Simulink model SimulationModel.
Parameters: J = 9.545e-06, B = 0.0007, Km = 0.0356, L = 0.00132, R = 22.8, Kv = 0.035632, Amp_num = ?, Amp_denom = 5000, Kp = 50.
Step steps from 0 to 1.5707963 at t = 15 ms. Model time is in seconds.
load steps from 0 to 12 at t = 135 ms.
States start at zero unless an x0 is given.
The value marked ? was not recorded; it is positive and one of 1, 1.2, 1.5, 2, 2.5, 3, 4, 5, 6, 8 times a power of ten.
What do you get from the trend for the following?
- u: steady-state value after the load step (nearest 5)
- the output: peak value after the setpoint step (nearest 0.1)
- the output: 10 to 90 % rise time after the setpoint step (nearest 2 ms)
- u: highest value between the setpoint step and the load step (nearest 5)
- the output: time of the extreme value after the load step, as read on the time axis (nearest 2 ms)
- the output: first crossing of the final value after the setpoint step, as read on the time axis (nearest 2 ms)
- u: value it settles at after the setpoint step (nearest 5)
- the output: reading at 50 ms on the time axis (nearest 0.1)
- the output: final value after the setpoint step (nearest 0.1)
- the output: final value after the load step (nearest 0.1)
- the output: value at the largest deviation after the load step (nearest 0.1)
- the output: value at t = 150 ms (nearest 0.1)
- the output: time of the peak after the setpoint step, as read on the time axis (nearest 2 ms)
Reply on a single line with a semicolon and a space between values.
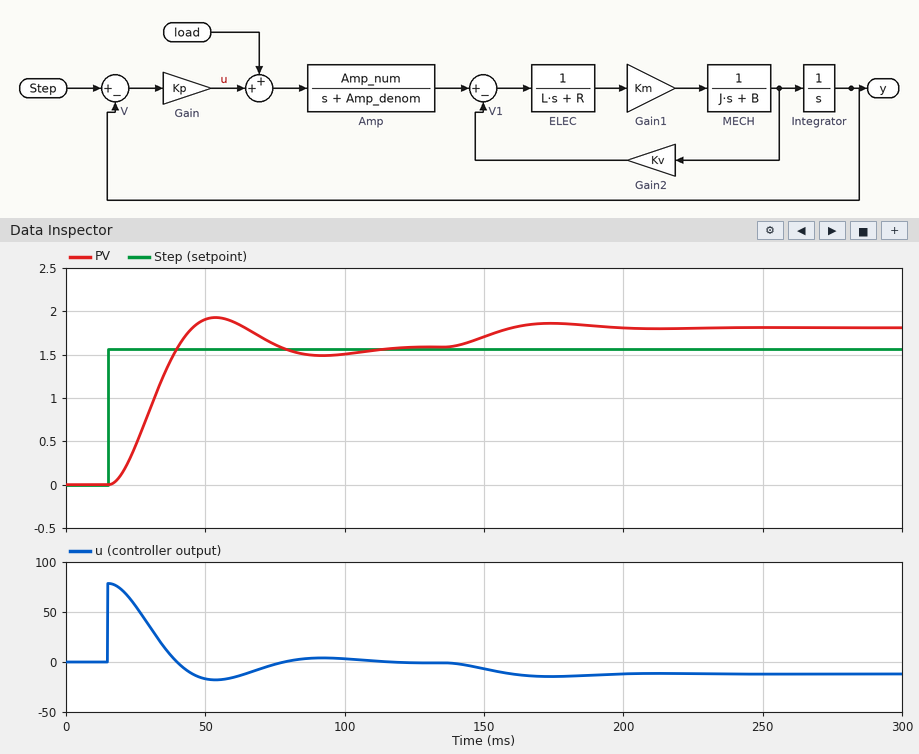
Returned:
-10; 1.9; 16 ms; 80; 174 ms; 40 ms; 0; 1.9; 1.6; 1.8; 1.9; 1.7; 54 ms
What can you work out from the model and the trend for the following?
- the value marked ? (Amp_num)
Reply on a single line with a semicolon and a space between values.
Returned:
5000
